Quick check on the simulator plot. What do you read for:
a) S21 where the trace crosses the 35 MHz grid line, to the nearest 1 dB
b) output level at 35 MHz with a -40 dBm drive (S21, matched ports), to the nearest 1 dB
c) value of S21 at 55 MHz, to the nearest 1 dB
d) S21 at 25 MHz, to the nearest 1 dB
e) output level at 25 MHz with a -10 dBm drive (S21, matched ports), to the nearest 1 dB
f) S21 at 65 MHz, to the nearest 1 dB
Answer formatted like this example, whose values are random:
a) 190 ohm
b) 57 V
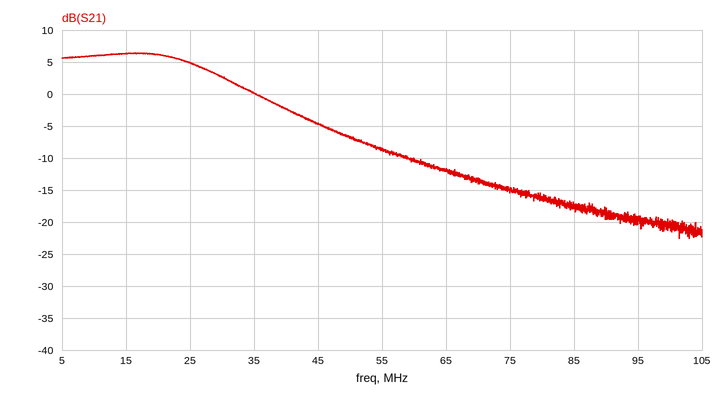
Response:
a) 0 dB
b) -40 dBm
c) -9 dB
d) 5 dB
e) -5 dBm
f) -12 dB
